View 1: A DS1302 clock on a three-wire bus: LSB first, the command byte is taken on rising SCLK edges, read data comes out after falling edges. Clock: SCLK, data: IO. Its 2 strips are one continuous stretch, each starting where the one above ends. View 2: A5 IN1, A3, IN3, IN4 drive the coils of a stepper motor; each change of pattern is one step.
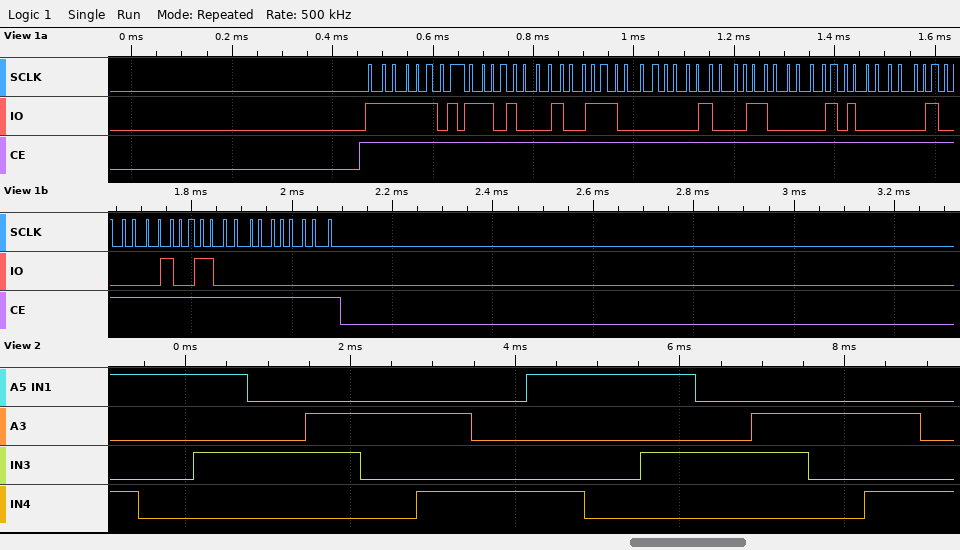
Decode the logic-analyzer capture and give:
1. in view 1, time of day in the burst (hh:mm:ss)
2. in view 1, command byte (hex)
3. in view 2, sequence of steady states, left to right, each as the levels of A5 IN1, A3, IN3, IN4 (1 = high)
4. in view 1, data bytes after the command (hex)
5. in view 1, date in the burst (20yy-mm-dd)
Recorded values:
20:39:17
0xBF
1001 1000 1010 0010 0110 0100 0101 0001 1001 1000 1010 0010 0110 0100 0101 0001
17 39 20 06 05 02 19 00
2019-05-06
